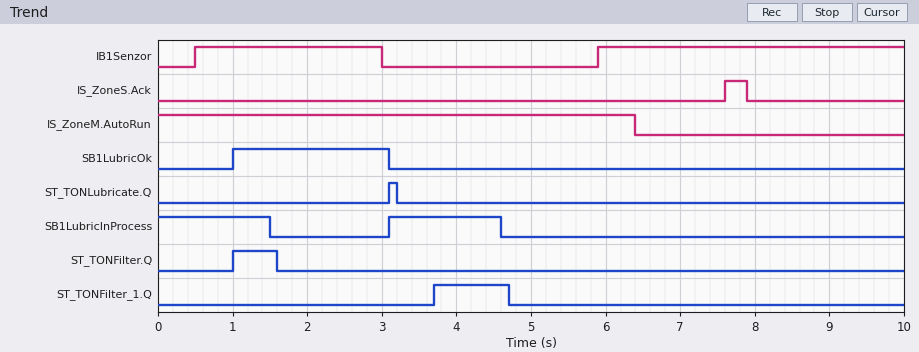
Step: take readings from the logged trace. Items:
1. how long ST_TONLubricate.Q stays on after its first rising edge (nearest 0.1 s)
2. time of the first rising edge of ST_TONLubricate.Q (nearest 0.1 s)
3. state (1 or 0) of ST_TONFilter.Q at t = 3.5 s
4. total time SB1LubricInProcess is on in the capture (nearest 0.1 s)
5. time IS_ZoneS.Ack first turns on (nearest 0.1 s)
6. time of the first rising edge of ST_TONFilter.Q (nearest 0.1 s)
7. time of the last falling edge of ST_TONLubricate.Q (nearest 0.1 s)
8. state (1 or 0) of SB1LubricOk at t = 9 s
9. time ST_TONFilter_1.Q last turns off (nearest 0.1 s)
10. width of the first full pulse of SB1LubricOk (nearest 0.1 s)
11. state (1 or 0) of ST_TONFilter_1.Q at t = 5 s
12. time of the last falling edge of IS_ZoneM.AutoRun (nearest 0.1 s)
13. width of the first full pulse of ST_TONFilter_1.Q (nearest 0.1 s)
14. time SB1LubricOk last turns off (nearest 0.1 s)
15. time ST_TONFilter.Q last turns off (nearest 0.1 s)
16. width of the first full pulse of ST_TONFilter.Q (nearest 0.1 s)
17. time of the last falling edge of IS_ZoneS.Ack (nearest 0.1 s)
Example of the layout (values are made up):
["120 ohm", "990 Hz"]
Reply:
["0.1 s", "3.1 s", "0", "3.0 s", "7.6 s", "1.0 s", "3.2 s", "0", "4.7 s", "2.1 s", "0", "6.4 s", "1.0 s", "3.1 s", "1.6 s", "0.6 s", "7.9 s"]
